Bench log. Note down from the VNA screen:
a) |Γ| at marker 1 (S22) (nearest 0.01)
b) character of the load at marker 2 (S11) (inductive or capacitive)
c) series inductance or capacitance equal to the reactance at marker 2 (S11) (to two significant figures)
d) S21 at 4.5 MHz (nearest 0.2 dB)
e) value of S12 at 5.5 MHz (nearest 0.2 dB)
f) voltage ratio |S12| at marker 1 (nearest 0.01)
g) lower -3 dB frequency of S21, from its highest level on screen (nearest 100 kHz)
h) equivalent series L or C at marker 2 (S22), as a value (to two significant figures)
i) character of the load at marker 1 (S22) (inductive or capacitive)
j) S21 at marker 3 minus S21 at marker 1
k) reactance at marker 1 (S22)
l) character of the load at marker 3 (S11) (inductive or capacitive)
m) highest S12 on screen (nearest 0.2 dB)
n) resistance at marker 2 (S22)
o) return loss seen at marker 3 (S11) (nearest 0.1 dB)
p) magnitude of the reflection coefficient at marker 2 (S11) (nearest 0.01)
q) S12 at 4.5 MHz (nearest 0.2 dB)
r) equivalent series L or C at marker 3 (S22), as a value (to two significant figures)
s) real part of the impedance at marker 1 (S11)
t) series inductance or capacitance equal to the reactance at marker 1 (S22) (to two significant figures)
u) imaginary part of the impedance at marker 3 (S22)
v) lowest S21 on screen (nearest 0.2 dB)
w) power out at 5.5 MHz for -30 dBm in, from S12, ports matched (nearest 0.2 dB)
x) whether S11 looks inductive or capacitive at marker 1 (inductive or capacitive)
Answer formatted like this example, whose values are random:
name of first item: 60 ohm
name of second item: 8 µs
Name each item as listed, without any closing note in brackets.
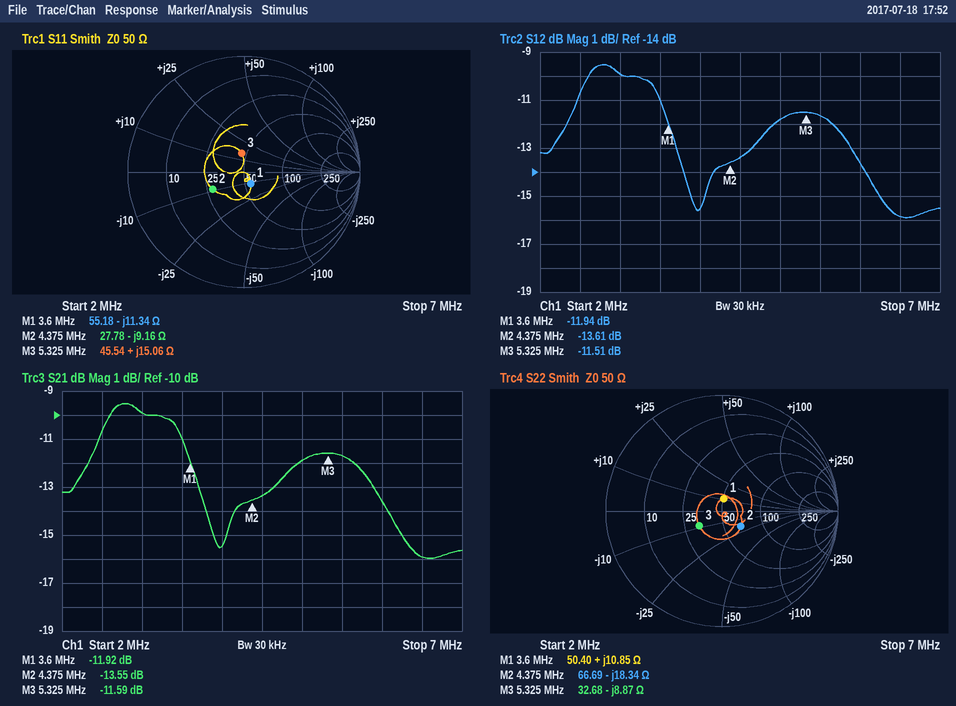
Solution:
|Γ| at marker 1 (S22): 0.11
character of the load at marker 2 (S11): capacitive
series inductance or capacitance equal to the reactance at marker 2 (S11): 4.0 nF
S21 at 4.5 MHz: -13.4 dB
value of S12 at 5.5 MHz: -11.6 dB
voltage ratio |S12| at marker 1: 0.25
lower -3 dB frequency of S21, from its highest level on screen: 2.2 MHz
equivalent series L or C at marker 2 (S22), as a value: 2.0 nF
character of the load at marker 1 (S22): inductive
S21 at marker 3 minus S21 at marker 1: 0.33 dB
reactance at marker 1: +10.85 Ω
character of the load at marker 3 (S11): inductive
highest S12 on screen: -9.6 dB
resistance at marker 2: 66.69 Ω
return loss seen at marker 3 (S11): 15.8 dB
magnitude of the reflection coefficient at marker 2 (S11): 0.31
S12 at 4.5 MHz: -13.4 dB
equivalent series L or C at marker 3 (S22), as a value: 3.4 nF
real part of the impedance at marker 1: 55.18 Ω
series inductance or capacitance equal to the reactance at marker 1 (S22): 480 nH
imaginary part of the impedance at marker 3: -8.87 Ω
lowest S21 on screen: -16.0 dB
power out at 5.5 MHz for -30 dBm in, from S12, ports matched: -41.6 dBm
whether S11 looks inductive or capacitive at marker 1: capacitive
